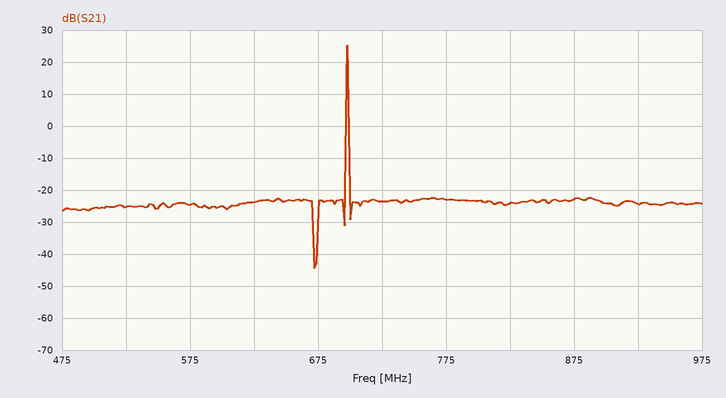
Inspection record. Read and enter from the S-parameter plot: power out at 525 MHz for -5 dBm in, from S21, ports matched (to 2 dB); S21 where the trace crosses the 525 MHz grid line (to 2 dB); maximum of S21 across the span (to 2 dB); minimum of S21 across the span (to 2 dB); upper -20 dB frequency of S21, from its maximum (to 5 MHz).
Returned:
-30 dBm
-26 dB
26 dB
-44 dB
700 MHz
